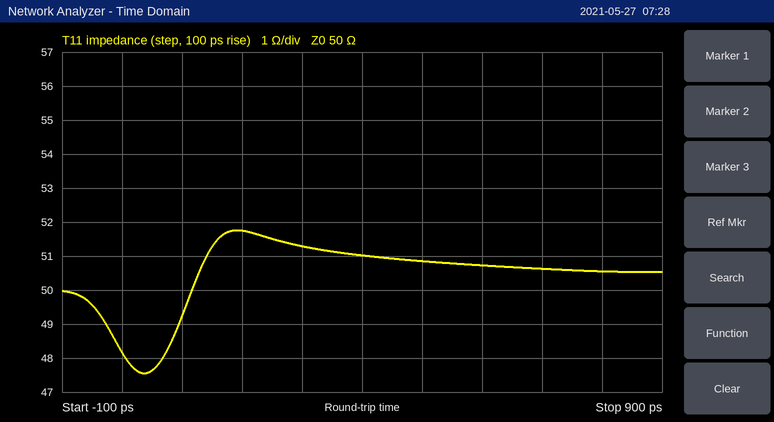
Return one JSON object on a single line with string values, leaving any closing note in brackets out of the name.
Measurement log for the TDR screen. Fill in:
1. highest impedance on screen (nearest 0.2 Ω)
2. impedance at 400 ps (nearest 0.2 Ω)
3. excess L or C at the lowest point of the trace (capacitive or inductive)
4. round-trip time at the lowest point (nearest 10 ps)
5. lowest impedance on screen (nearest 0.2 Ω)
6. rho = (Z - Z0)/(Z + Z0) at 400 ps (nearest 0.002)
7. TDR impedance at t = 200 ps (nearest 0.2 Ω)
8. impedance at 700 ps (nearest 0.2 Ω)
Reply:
{"highest impedance on screen": "51.8 Ω", "impedance at 400 ps": "51.0 Ω", "excess L or C at the lowest point of the trace": "capacitive", "round-trip time at the lowest point": "40 ps", "lowest impedance on screen": "47.6 Ω", "rho = (Z - Z0)/(Z + Z0) at 400 ps": "+0.010", "TDR impedance at t = 200 ps": "51.8 Ω", "impedance at 700 ps": "50.6 Ω"}
